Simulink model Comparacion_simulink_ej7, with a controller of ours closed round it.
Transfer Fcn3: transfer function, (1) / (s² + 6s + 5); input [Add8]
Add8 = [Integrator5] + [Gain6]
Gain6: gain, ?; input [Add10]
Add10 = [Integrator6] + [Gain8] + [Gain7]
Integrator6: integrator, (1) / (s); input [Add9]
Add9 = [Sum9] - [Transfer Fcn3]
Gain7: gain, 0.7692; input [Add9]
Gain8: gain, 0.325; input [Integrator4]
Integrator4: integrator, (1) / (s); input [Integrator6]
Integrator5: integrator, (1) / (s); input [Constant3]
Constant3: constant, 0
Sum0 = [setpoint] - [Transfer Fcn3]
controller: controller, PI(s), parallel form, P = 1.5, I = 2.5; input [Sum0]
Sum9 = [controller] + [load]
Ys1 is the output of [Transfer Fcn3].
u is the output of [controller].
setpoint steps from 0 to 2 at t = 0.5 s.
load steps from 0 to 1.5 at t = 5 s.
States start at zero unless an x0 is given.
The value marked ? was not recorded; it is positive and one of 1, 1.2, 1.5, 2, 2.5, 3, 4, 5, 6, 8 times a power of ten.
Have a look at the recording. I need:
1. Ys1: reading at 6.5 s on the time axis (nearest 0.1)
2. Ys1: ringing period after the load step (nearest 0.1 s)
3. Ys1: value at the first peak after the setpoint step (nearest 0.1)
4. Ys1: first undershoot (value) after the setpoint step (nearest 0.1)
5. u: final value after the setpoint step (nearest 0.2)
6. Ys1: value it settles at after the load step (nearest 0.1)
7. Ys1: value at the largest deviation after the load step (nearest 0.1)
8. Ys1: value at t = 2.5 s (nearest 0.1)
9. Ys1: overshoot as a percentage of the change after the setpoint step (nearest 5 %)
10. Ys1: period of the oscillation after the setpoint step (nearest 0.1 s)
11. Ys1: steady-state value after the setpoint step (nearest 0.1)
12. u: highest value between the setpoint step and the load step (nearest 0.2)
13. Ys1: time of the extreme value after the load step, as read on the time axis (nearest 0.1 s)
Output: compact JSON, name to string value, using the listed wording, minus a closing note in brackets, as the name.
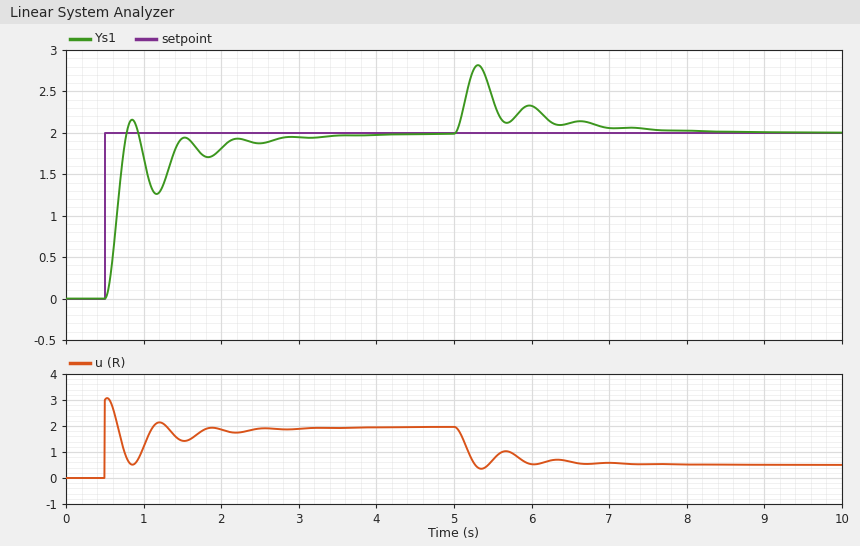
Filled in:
{"Ys1: reading at 6.5 s on the time axis": "2.1", "Ys1: ringing period after the load step": "0.7 s", "Ys1: value at the first peak after the setpoint step": "2.2", "Ys1: first undershoot (value) after the setpoint step": "1.3", "u: final value after the setpoint step": "2.0", "Ys1: value it settles at after the load step": "2.0", "Ys1: value at the largest deviation after the load step": "2.8", "Ys1: value at t = 2.5 s": "1.9", "Ys1: overshoot as a percentage of the change after the setpoint step": "10 %", "Ys1: period of the oscillation after the setpoint step": "0.7 s", "Ys1: steady-state value after the setpoint step": "2.0", "u: highest value between the setpoint step and the load step": "3.0", "Ys1: time of the extreme value after the load step, as read on the time axis": "5.3 s"}
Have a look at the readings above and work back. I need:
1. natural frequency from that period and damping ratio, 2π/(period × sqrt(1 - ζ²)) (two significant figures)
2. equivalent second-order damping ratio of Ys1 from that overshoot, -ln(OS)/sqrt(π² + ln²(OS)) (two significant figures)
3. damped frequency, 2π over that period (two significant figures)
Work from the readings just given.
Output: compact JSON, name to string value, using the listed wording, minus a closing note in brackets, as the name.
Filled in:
{"natural frequency from that period and damping ratio, 2π/(period × sqrt(1 - ζ²))": "11 rad/s", "equivalent second-order damping ratio of Ys1 from that overshoot, -ln(OS)/sqrt(π² + ln²(OS))": "0.59", "damped frequency, 2π over that period": "9.0 rad/s"}
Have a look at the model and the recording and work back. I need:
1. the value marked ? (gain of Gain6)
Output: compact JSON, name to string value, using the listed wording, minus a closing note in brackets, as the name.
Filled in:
{"the value marked ?": "50"}
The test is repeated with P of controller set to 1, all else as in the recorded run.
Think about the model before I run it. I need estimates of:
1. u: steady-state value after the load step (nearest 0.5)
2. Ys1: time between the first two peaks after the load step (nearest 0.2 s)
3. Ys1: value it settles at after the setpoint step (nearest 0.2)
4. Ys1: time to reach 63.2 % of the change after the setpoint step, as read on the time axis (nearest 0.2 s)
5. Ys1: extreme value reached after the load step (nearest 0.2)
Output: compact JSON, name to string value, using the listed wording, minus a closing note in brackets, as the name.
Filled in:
{"u: steady-state value after the load step": "0.5", "Ys1: time between the first two peaks after the load step": "0.8 s", "Ys1: value it settles at after the setpoint step": "2.0", "Ys1: time to reach 63.2 % of the change after the setpoint step, as read on the time axis": "0.8 s", "Ys1: extreme value reached after the load step": "3.0"}
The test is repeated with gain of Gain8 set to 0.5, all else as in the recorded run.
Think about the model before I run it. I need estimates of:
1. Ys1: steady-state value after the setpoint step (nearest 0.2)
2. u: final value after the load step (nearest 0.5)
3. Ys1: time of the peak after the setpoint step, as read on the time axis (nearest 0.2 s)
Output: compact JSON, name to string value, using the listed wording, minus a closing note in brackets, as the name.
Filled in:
{"Ys1: steady-state value after the setpoint step": "2.0", "u: final value after the load step": "0.5", "Ys1: time of the peak after the setpoint step, as read on the time axis": "0.8 s"}
